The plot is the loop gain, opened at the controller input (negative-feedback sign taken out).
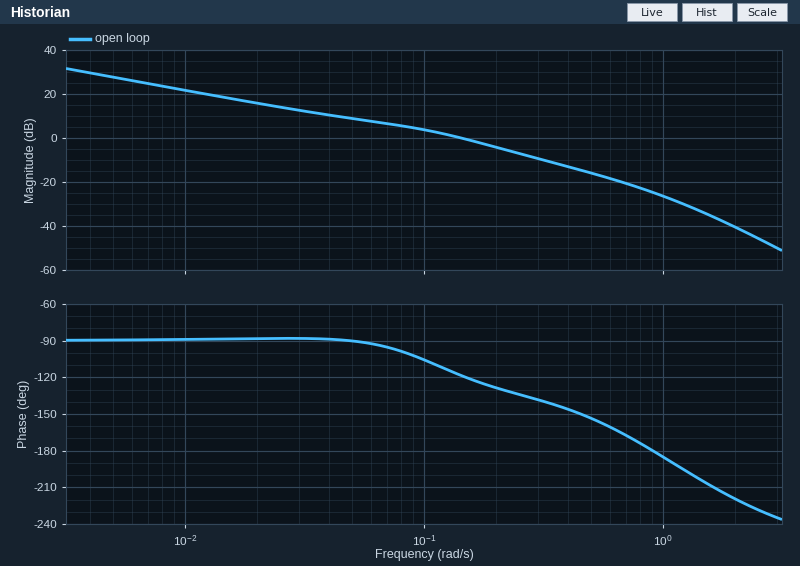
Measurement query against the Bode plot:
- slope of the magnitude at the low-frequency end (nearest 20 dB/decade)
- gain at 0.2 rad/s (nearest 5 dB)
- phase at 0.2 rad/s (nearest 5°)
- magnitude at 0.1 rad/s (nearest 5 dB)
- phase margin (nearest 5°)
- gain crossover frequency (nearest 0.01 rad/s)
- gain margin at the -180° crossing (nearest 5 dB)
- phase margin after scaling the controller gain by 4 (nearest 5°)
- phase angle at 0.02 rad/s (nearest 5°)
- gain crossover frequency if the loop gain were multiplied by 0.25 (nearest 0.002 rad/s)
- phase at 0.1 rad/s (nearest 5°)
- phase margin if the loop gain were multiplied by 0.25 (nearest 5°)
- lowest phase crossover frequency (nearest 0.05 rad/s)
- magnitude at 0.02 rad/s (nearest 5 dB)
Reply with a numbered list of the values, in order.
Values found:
1. -20 dB/decade
2. -5 dB
3. -130°
4. 5 dB
5. 60°
6. 0.14 rad/s
7. 25 dB
8. 35°
9. -90°
10. 0.032 rad/s
11. -105°
12. 90°
13. 0.90 rad/s
14. 15 dB
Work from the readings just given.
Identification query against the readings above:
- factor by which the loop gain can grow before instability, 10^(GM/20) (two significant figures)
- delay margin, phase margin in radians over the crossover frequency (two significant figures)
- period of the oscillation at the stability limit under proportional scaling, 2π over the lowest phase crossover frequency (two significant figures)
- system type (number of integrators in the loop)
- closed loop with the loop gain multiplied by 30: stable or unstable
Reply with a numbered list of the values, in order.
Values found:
1. 18
2. 7.5 s
3. 7.0 s
4. 1
5. unstable
